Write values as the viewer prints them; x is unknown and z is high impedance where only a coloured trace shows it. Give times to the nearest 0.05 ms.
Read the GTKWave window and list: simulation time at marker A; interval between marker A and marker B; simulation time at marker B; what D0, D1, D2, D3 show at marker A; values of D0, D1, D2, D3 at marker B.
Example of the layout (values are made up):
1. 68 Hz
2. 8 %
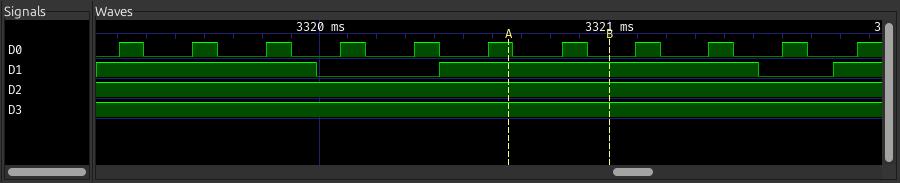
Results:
1. 3320.65 ms
2. 0.35 ms
3. 3321 ms
4. D0=1, D1=1, D2=1, D3=1
5. D0=0, D1=1, D2=1, D3=1
